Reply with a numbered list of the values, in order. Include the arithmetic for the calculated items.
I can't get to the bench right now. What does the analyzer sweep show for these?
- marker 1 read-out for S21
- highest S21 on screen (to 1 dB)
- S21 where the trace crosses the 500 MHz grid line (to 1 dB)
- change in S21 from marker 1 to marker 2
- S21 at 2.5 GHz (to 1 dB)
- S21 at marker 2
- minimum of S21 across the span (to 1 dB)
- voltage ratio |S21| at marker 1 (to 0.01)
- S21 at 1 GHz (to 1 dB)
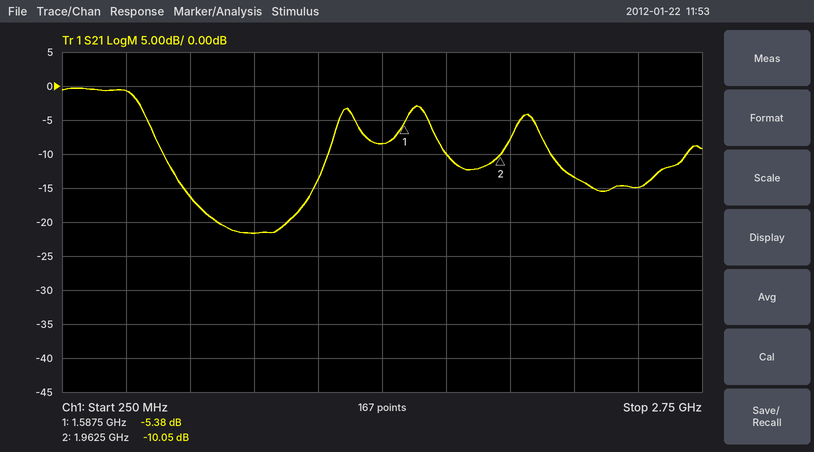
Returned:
1. -5.38 dB
2. 0 dB
3. -1 dB
4. -10.05 − (-5.38) = -4.67 dB
5. -15 dB
6. -10.05 dB
7. -22 dB
8. 10^(-5.38/20) ≈ 0.54
9. -22 dB
